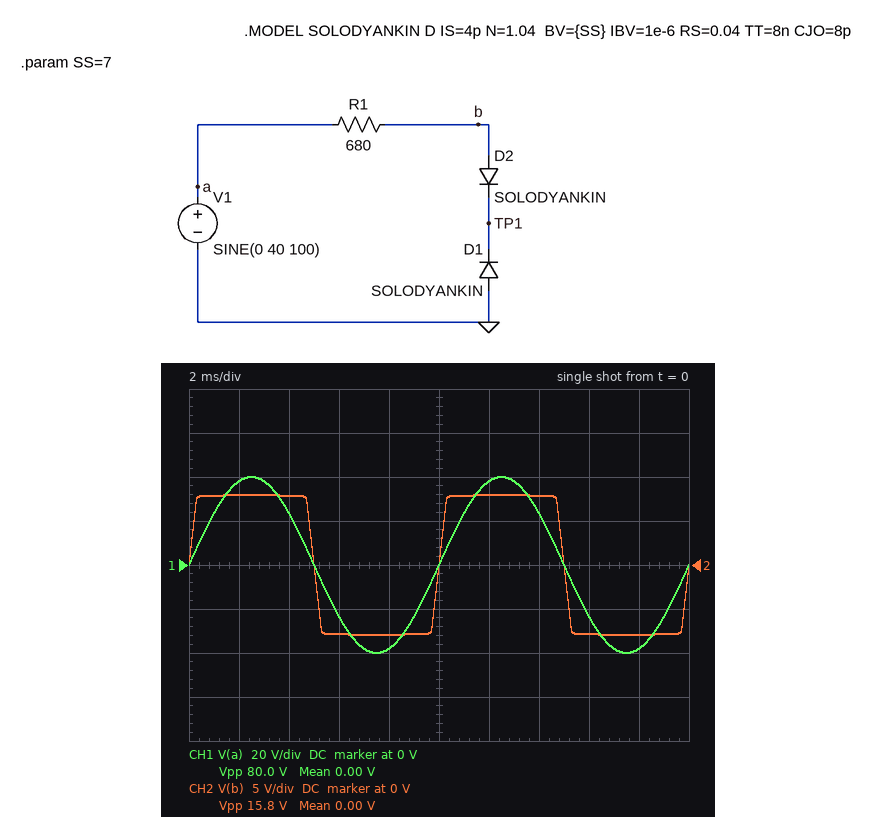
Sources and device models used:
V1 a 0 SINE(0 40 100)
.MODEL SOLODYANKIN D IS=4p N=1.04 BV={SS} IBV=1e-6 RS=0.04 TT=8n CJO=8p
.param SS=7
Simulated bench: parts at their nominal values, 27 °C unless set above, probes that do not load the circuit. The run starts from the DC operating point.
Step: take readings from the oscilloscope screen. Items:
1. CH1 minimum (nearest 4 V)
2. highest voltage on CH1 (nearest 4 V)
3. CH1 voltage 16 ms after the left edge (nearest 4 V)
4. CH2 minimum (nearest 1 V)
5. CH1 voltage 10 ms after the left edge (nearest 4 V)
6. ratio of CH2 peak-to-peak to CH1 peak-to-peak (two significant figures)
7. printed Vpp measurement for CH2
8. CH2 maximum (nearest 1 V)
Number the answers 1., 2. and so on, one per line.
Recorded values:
1. -40 V
2. 40 V
3. -24 V
4. -8 V
5. 0 V
6. 0.20
7. 15.8 V
8. 8 V
